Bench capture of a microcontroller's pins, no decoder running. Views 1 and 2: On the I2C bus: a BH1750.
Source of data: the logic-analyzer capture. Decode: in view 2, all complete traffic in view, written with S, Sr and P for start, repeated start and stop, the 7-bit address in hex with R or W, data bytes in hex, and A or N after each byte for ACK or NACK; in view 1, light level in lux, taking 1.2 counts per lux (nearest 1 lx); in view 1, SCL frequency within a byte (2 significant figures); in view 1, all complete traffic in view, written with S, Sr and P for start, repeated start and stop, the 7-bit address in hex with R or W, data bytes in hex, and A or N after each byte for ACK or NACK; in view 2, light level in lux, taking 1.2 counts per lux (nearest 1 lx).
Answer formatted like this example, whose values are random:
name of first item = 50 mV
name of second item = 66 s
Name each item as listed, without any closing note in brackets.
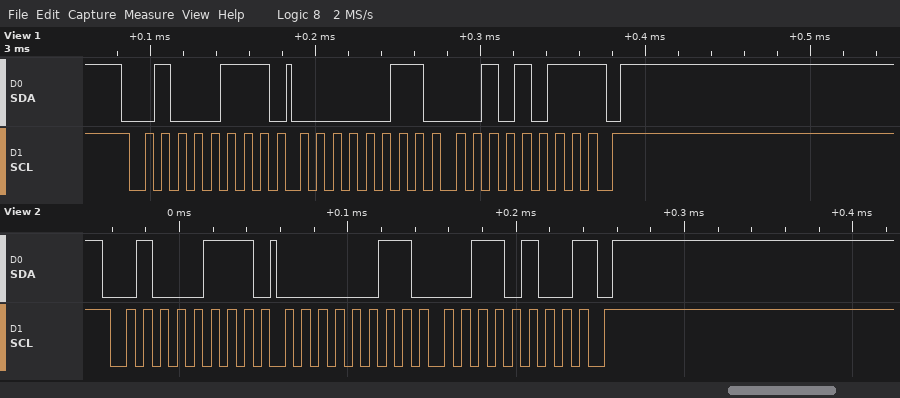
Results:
in view 2, all complete traffic in view, written with S, Sr and P for start, repeated start and stop, the 7-bit address in hex with R or W, data bytes in hex, and A or N after each byte for ACK or NACK = S 23R A 03 A 34 N P
in view 1, light level in lux, taking 1.2 counts per lux = 676 lx
in view 1, SCL frequency within a byte = 100 kHz
in view 1, all complete traffic in view, written with S, Sr and P for start, repeated start and stop, the 7-bit address in hex with R or W, data bytes in hex, and A or N after each byte for ACK or NACK = S 23R A 03 A 2B N P
in view 2, light level in lux, taking 1.2 counts per lux = 683 lx
